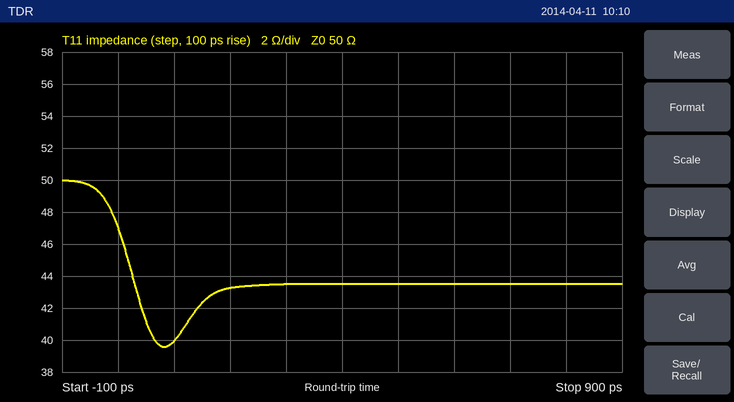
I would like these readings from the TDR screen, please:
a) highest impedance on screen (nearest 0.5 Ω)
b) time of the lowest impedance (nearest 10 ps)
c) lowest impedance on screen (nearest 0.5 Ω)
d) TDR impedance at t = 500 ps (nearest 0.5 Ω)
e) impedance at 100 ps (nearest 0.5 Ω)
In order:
50.0 Ω
80 ps
39.5 Ω
43.5 Ω
40.0 Ω
